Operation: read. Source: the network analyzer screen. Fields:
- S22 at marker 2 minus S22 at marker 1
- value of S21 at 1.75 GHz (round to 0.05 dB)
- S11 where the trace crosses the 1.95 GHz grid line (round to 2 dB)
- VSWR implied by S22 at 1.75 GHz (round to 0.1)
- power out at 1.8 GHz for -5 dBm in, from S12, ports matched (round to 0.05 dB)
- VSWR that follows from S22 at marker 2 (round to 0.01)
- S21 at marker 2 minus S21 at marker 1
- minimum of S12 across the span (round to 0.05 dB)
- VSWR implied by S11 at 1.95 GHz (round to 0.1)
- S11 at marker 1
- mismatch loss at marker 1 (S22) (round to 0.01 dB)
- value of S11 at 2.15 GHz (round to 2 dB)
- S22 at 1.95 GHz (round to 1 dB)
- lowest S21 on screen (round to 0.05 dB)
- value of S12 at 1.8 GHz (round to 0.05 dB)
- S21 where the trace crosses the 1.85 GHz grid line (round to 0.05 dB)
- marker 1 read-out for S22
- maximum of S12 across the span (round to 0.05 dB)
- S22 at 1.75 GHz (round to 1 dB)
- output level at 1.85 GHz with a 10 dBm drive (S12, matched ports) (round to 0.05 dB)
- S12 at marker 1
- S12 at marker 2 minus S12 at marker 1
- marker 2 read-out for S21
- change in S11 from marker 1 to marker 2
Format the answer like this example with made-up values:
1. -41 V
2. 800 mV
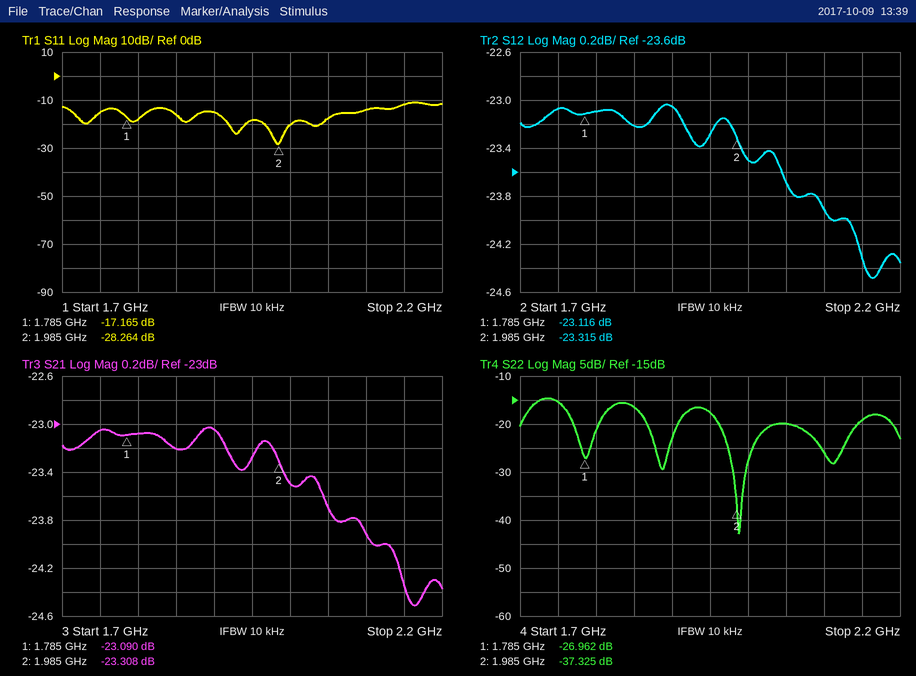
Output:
1. -10.363 dB
2. -23.05 dB
3. -18 dB
4. 1.4
5. -28.10 dBm
6. 1.03
7. -0.218 dB
8. -24.50 dB
9. 1.3
10. -17.165 dB
11. 0.01 dB
12. -12 dB
13. -18 dB
14. -24.50 dB
15. -23.10 dB
16. -23.20 dB
17. -26.962 dB
18. -23.05 dB
19. -15 dB
20. -13.20 dBm
21. -23.116 dB
22. -0.199 dB
23. -23.308 dB
24. -11.099 dB
